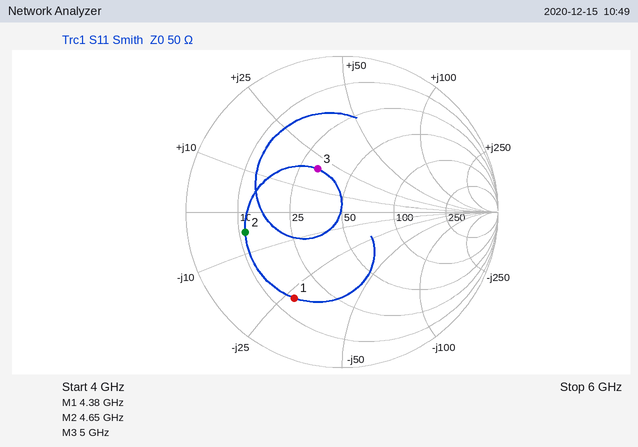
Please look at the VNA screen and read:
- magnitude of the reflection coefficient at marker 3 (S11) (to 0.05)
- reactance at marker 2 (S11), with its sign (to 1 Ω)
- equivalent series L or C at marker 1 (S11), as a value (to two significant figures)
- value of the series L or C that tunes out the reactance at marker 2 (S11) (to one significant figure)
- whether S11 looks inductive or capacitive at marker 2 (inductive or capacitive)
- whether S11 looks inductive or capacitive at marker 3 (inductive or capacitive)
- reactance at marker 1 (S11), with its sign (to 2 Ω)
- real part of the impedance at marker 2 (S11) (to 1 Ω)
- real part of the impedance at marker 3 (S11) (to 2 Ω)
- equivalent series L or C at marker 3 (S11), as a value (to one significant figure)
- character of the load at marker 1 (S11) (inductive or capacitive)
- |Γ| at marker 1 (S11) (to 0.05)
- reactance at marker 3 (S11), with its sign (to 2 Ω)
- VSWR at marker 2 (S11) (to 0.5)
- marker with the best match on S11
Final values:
0.30
-5 Ω
1.3 pF
200 pH
capacitive
inductive
-28 Ω
11 Ω
32 Ω
600 pH
capacitive
0.65
+20 Ω
4.5
marker 3
